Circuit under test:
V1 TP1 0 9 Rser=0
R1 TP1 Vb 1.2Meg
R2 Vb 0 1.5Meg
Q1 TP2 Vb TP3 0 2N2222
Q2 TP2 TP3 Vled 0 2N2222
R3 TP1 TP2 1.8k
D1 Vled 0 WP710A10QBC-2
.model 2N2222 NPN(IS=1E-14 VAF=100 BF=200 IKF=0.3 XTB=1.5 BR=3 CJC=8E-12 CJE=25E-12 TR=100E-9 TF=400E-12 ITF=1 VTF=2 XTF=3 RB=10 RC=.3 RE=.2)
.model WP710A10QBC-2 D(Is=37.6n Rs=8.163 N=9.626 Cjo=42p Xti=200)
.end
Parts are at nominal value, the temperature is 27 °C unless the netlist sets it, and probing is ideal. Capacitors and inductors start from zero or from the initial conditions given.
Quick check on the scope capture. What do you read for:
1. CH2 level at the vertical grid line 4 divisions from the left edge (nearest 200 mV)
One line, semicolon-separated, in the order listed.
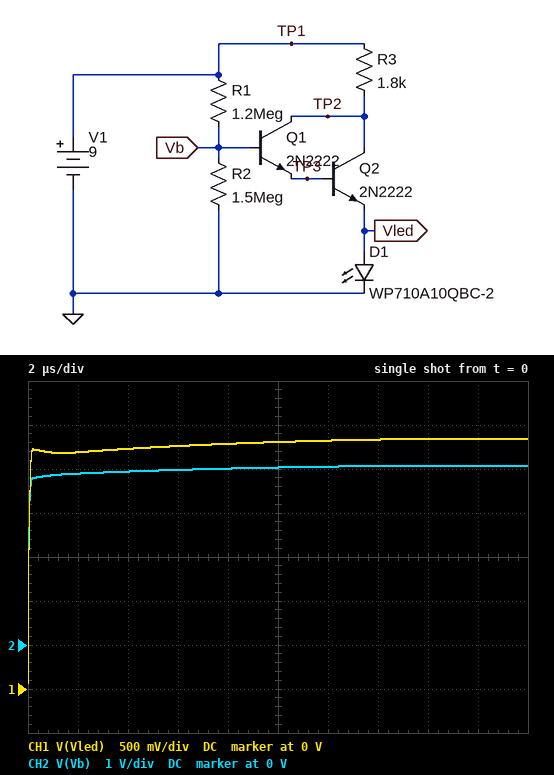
4.0 V
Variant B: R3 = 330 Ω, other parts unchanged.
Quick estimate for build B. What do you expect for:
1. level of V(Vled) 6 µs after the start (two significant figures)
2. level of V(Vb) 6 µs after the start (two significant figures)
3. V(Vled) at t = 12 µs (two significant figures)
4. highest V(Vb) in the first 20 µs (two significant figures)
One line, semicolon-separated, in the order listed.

3.1 V; 4.4 V; 3.2 V; 4.5 V
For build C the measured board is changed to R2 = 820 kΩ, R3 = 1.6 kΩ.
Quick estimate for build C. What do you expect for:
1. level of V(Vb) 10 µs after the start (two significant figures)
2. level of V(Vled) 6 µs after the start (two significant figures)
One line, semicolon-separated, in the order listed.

3.8 V; 2.6 V
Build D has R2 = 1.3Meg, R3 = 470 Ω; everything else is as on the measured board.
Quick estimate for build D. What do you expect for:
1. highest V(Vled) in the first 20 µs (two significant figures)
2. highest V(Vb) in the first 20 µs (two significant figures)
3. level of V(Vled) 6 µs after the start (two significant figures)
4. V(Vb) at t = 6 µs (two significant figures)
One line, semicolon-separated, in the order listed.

3.1 V; 4.4 V; 3.0 V; 4.3 V
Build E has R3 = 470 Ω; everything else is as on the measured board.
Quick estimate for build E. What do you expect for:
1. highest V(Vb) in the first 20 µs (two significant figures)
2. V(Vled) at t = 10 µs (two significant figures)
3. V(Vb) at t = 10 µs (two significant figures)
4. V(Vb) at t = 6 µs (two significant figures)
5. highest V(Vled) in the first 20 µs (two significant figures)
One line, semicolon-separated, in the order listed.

4.5 V; 3.1 V; 4.4 V; 4.3 V; 3.2 V
